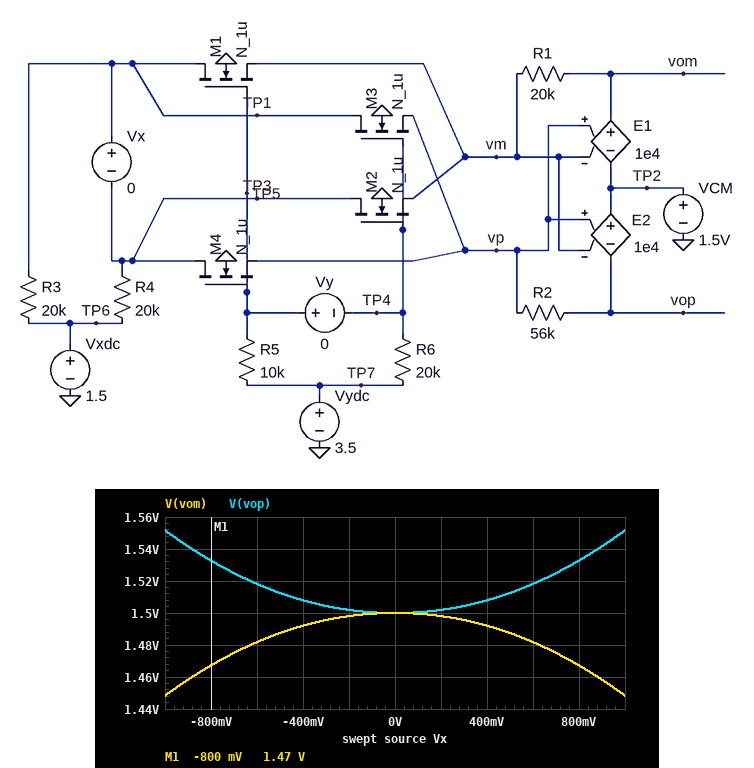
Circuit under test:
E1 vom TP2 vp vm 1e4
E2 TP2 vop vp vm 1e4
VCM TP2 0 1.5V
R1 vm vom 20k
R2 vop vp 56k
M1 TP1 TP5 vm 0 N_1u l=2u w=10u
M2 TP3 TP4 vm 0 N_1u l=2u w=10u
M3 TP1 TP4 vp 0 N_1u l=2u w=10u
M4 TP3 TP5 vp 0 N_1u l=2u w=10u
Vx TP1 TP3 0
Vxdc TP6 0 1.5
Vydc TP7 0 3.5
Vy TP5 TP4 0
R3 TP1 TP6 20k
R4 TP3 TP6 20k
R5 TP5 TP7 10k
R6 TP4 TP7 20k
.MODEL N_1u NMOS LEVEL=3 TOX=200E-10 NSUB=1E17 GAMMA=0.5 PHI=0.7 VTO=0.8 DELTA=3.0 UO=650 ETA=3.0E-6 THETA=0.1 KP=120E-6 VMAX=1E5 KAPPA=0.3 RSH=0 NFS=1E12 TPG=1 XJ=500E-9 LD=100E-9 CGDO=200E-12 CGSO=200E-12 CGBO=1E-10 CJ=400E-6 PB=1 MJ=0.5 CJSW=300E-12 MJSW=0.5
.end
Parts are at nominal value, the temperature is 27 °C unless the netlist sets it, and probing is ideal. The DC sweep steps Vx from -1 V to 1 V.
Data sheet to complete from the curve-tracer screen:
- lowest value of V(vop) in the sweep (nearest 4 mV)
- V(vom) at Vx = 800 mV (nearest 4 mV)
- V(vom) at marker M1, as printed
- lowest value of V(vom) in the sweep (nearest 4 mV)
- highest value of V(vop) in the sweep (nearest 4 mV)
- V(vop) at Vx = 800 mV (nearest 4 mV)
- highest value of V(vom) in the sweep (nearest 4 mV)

1.500 V
1.468 V
1.47 V
1.448 V
1.552 V
1.532 V
1.500 V
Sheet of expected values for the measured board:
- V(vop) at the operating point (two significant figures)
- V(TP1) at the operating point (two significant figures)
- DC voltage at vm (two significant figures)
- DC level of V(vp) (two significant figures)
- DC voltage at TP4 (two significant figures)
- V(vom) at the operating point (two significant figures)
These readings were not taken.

1.5 V
1.5 V
1.5 V
1.5 V
3.5 V
1.5 V
